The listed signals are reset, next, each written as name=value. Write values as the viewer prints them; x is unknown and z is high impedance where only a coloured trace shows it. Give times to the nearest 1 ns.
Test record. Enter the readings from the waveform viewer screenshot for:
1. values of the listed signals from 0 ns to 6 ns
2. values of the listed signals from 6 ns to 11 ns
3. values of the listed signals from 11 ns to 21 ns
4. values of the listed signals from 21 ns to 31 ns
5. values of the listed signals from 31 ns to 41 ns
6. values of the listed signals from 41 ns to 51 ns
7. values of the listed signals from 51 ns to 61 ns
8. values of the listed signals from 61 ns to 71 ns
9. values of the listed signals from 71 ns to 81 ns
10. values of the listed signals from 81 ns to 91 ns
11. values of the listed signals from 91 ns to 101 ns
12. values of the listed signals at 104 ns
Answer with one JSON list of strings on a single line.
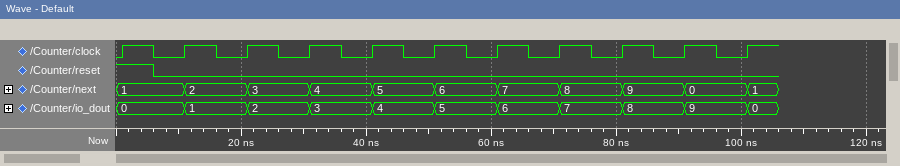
["reset=1, next=1", "reset=0, next=1", "reset=0, next=2", "reset=0, next=3", "reset=0, next=4", "reset=0, next=5", "reset=0, next=6", "reset=0, next=7", "reset=0, next=8", "reset=0, next=9", "reset=0, next=0", "reset=0, next=1"]
